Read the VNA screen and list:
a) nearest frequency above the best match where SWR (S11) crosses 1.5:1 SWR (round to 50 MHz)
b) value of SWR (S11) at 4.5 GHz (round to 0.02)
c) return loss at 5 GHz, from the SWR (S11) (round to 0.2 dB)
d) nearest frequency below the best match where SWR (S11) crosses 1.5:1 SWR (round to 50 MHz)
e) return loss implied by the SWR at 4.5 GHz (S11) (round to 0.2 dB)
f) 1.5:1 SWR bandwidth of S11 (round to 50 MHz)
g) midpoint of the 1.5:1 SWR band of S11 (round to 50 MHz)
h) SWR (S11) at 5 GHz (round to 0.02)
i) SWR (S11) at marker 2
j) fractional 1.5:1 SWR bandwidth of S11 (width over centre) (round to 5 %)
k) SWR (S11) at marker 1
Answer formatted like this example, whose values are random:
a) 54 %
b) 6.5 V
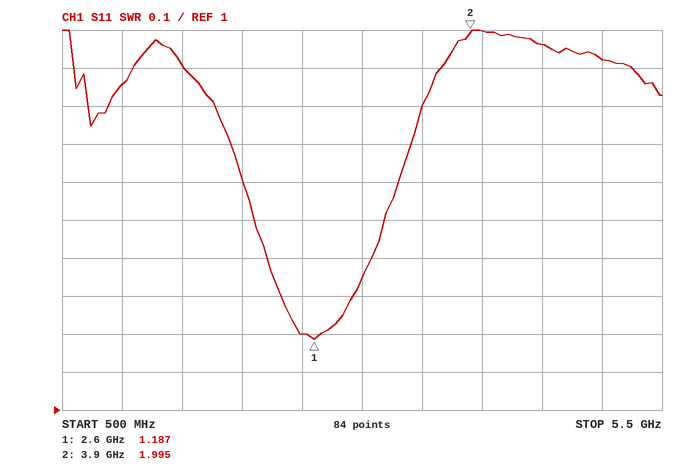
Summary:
a) 3.20 GHz
b) 1.96
c) 10.0 dB
d) 2.10 GHz
e) 9.8 dB
f) 1.10 GHz
g) 2.65 GHz
h) 1.92
i) 1.995
j) 40 %
k) 1.187
